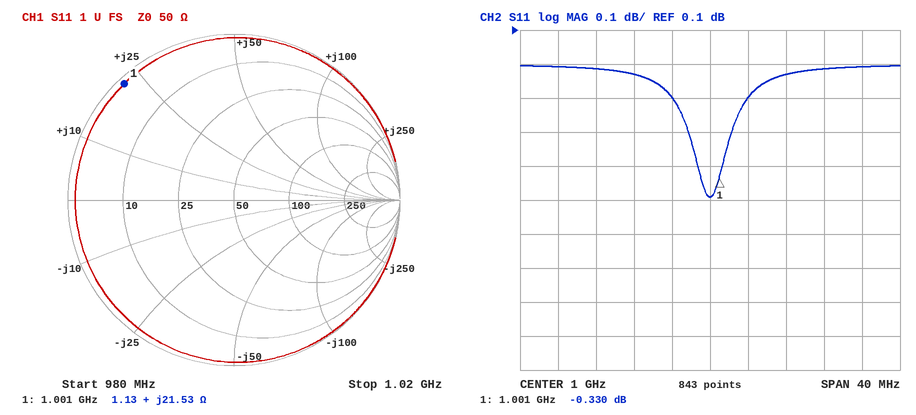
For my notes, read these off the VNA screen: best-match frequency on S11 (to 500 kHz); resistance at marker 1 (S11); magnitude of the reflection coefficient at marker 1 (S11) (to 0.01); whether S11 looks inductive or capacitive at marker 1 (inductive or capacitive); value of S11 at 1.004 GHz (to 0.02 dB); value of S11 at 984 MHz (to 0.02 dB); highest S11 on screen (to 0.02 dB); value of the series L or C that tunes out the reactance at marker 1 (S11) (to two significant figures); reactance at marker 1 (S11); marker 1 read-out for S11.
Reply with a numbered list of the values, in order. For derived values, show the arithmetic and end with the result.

1. 1.0000 GHz
2. 1.13 Ω
3. 0.96
4. inductive
5. -0.10 dB
6. 0.00 dB
7. 0.00 dB
8. C = 1/(2π × 1.001 GHz × 21.53 Ω) ≈ 7.4 pF
9. +21.53 Ω
10. -0.330 dB
